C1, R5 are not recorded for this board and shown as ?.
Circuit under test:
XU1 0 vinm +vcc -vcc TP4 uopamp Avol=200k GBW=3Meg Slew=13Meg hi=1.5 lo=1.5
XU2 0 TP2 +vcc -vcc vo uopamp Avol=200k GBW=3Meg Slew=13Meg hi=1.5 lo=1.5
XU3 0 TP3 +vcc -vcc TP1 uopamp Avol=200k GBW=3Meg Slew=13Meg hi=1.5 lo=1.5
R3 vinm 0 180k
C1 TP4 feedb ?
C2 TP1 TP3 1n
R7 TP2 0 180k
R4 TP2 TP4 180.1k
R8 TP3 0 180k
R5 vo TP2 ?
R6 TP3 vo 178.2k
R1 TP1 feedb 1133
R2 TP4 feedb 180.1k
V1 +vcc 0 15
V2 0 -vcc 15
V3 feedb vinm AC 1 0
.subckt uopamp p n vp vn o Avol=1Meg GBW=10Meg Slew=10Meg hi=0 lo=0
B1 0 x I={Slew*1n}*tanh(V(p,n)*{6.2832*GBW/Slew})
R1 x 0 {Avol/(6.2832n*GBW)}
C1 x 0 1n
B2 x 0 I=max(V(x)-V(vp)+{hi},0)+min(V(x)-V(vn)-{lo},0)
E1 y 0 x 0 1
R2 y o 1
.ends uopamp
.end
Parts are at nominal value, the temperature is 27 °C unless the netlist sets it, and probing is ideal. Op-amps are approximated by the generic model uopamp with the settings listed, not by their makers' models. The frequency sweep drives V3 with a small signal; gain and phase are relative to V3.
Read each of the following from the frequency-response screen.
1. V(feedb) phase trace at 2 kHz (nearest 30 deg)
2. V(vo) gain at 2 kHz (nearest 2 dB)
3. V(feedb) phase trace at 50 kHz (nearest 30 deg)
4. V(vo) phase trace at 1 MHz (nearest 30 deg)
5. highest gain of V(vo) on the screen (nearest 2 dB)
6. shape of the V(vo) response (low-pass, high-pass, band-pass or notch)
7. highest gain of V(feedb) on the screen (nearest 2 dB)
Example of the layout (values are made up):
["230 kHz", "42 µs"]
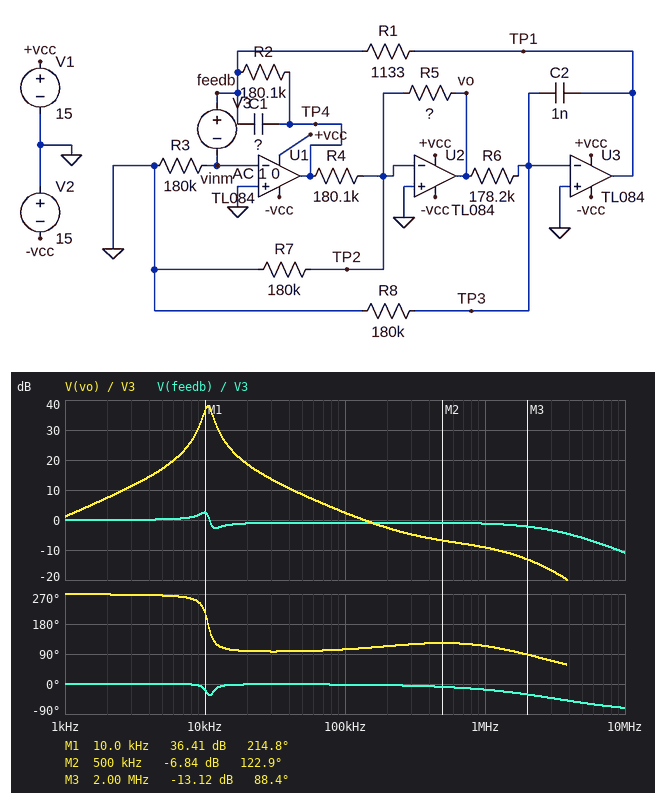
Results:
["0 deg", "8 dB", "0 deg", "120 deg", "38 dB", "band-pass", "2 dB"]
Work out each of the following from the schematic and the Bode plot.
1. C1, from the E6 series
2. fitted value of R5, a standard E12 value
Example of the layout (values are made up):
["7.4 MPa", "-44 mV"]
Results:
["470 pF", "82 kΩ"]
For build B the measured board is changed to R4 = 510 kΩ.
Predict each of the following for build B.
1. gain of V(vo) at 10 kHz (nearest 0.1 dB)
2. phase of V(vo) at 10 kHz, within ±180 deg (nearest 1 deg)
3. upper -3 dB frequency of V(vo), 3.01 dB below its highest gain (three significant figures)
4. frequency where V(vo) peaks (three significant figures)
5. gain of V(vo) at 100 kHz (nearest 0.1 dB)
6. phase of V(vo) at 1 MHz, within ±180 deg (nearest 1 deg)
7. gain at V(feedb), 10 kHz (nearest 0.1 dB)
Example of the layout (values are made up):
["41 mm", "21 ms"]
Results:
["16.8 dB", "107 deg", "7.13 kHz", "6.24 kHz", "-6.7 dB", "118 deg", "-1.3 dB"]
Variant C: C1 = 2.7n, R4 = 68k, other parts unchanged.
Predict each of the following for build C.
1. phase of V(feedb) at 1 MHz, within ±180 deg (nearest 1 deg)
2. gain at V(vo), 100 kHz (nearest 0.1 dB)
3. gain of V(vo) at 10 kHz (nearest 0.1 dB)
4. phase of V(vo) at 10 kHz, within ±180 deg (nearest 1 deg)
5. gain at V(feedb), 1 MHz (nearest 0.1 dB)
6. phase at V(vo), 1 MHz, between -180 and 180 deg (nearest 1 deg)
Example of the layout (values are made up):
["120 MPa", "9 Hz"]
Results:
["-18 deg", "2.5 dB", "22.9 dB", "103 deg", "-0.6 dB", "117 deg"]
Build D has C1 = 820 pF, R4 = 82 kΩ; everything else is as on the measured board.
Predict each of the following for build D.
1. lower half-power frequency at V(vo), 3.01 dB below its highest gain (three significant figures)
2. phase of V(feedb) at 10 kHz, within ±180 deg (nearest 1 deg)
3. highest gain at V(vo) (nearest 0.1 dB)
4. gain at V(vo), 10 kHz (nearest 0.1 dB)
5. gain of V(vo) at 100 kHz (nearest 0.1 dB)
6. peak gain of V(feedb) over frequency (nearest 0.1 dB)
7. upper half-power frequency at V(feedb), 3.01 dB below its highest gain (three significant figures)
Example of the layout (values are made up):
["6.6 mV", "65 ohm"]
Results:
["11.6 kHz", "-1 deg", "46.1 dB", "31.1 dB", "5.6 dB", "3.5 dB", "12.2 kHz"]
